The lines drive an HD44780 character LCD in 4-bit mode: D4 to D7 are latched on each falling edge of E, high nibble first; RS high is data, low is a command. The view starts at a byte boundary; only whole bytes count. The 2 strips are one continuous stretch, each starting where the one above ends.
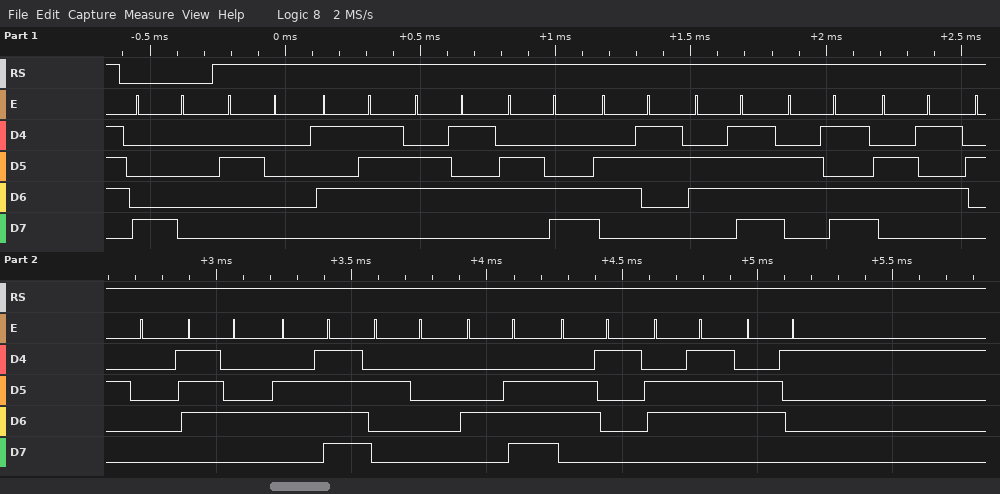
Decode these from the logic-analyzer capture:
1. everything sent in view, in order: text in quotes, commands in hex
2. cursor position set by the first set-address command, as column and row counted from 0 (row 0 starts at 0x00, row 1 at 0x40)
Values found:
0x80 " Welcome to Naga"
column 0, row 0
